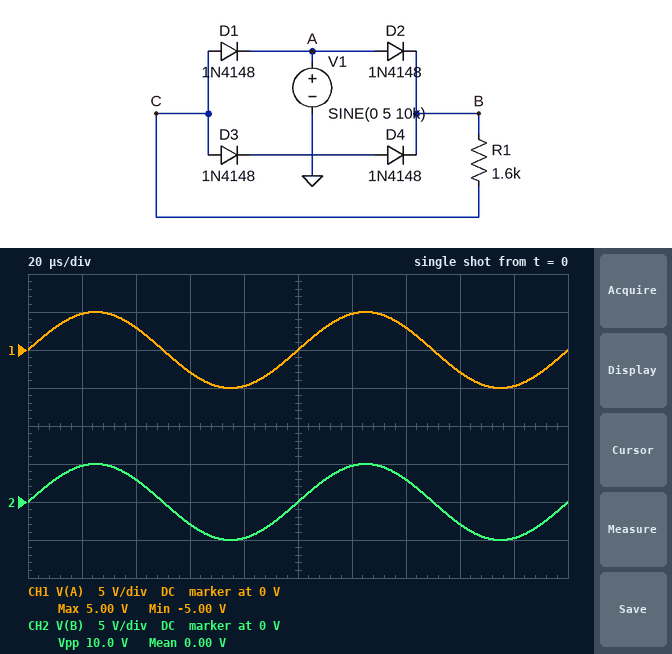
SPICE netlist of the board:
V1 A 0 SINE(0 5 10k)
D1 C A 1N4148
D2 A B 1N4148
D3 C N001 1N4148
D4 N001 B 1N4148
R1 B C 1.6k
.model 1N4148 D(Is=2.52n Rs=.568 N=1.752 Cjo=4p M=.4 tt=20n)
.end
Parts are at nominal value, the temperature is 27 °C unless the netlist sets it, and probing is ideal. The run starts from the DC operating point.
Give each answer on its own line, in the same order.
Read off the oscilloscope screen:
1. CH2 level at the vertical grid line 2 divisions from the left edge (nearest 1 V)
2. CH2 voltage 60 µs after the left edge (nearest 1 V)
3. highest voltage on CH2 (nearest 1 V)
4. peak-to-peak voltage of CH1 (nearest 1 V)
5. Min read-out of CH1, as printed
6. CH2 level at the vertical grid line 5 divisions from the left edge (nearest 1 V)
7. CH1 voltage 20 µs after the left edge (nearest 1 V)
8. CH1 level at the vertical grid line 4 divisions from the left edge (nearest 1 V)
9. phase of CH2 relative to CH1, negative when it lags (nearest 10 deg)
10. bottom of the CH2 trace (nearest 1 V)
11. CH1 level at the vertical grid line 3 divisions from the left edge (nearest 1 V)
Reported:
3 V
-3 V
5 V
10 V
-5.00 V
0 V
5 V
-5 V
0 deg
-5 V
-3 V
